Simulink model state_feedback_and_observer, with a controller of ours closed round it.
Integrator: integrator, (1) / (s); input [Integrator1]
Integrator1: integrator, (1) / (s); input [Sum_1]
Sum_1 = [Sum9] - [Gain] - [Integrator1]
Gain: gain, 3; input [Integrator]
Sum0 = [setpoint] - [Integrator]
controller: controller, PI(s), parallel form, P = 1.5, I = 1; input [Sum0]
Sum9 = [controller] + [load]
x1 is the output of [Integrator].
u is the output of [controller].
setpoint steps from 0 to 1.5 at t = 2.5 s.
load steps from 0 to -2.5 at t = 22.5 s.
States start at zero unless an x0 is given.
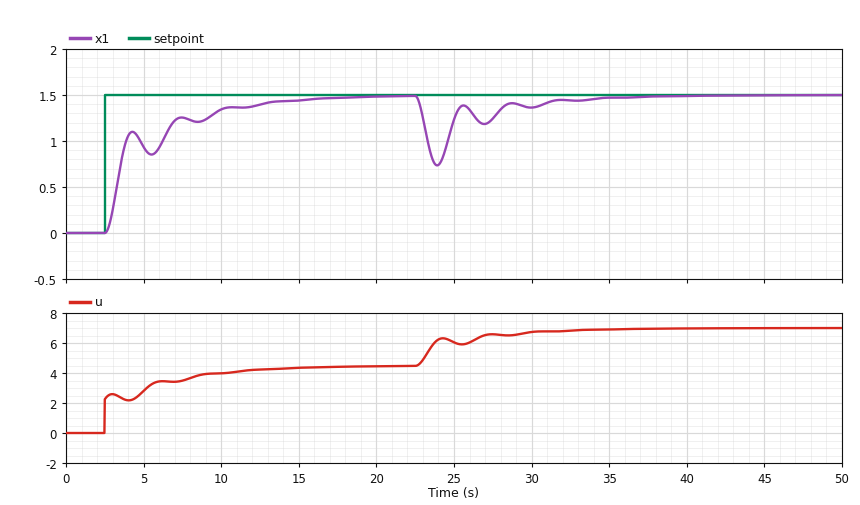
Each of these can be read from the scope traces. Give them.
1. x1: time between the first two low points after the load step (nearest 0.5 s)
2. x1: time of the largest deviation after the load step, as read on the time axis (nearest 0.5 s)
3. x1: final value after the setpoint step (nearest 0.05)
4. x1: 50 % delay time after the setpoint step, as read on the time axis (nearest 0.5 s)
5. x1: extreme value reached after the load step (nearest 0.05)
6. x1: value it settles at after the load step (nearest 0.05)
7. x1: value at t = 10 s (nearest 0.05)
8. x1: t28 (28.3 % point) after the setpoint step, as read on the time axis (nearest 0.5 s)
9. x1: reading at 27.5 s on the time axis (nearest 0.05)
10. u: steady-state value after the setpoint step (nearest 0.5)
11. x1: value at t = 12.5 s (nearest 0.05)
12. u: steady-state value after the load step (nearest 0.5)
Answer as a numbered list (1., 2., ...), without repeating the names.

1. 3.0 s
2. 24.0 s
3. 1.50
4. 3.5 s
5. 0.75
6. 1.50
7. 1.35
8. 3.0 s
9. 1.25
10. 4.5
11. 1.40
12. 7.0
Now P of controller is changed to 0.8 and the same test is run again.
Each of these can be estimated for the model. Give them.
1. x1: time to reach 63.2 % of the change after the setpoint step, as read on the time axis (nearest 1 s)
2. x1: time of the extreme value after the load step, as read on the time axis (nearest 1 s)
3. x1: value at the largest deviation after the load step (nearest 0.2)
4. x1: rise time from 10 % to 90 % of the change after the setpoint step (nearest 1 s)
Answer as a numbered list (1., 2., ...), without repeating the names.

1. 4 s
2. 24 s
3. 0.6
4. 7 s
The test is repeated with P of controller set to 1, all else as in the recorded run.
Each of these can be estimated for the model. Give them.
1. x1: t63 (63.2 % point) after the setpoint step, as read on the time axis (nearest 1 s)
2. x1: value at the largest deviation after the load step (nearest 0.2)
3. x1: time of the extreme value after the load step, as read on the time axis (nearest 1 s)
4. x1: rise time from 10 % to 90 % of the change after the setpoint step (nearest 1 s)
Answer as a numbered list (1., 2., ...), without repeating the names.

1. 4 s
2. 0.6
3. 24 s
4. 7 s
